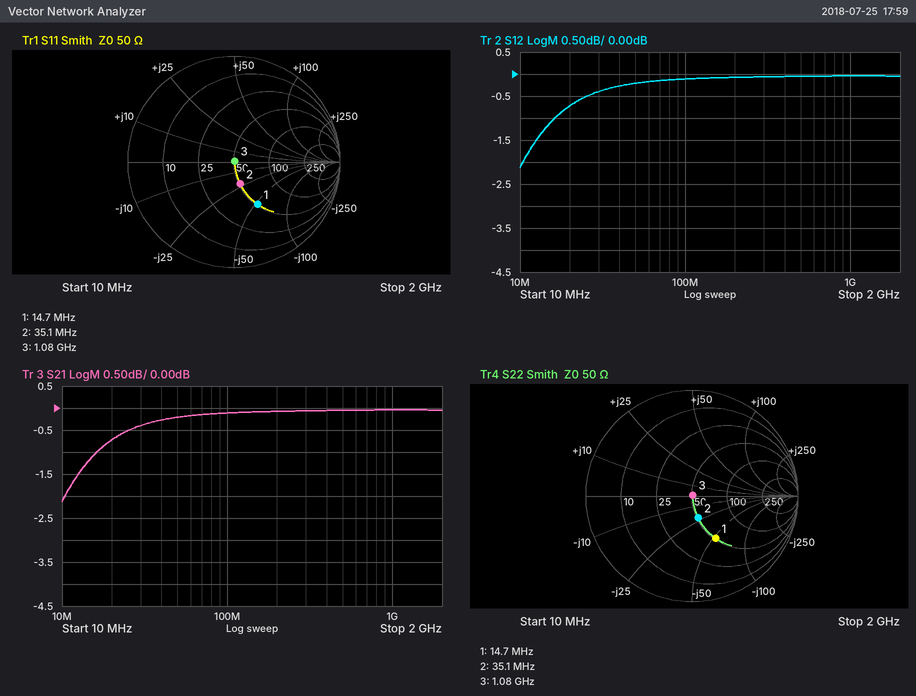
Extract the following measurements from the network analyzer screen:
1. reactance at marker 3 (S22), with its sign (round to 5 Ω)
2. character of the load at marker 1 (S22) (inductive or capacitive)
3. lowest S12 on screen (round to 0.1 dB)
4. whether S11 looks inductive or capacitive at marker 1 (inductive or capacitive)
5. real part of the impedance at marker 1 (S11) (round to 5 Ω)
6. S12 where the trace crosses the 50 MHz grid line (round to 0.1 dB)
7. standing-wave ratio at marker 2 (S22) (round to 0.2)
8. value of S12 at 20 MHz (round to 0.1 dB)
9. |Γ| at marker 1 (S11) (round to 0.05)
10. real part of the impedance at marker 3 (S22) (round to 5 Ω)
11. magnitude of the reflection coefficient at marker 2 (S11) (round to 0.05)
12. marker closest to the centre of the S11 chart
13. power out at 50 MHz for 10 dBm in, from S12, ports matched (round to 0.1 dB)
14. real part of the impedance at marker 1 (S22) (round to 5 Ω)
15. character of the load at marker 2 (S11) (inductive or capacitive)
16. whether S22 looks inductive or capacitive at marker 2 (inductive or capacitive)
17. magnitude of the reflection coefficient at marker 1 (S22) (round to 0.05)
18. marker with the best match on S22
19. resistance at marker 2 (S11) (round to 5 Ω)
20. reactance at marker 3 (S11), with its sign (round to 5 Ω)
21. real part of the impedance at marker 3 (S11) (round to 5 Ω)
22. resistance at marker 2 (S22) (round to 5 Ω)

0 Ω
capacitive
-2.1 dB
capacitive
50 Ω
-0.2 dB
1.6
-0.7 dB
0.45
50 Ω
0.20
marker 3
9.8 dBm
50 Ω
capacitive
capacitive
0.45
marker 3
50 Ω
0 Ω
50 Ω
50 Ω
